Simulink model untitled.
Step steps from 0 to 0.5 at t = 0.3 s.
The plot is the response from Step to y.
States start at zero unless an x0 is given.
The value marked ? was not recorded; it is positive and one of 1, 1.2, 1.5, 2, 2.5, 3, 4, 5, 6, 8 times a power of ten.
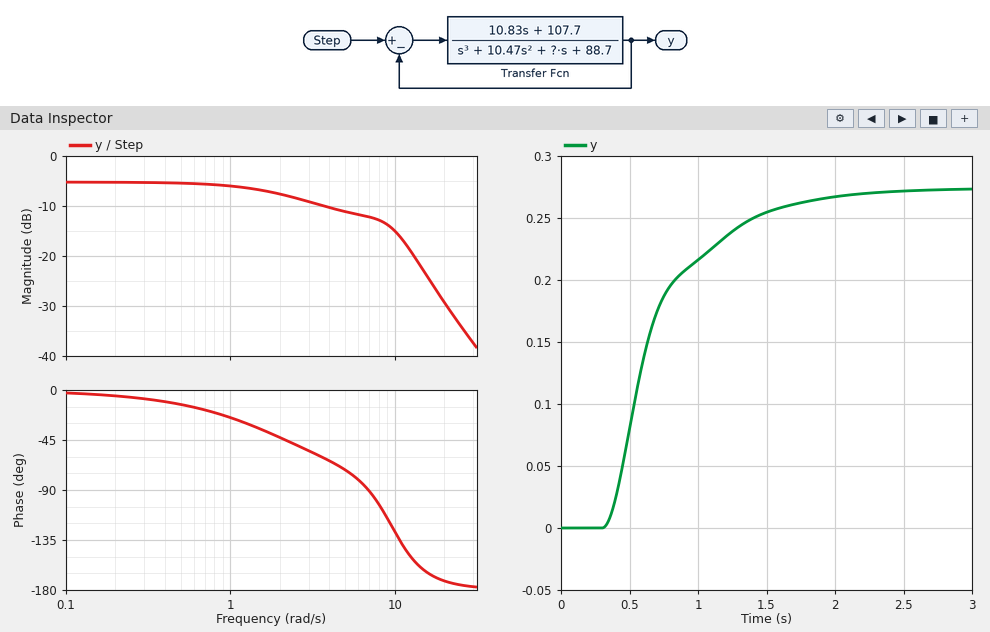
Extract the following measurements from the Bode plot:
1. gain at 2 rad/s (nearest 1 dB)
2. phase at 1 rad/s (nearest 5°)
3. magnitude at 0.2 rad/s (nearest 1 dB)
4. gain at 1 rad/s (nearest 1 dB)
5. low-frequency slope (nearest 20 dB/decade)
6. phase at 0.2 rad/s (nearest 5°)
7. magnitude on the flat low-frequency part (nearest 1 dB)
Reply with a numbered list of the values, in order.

1. -8 dB
2. -25°
3. -5 dB
4. -6 dB
5. 0 dB/decade
6. -5°
7. -5 dB
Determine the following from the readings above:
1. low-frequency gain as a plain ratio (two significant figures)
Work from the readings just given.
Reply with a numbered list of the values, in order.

1. 0.56
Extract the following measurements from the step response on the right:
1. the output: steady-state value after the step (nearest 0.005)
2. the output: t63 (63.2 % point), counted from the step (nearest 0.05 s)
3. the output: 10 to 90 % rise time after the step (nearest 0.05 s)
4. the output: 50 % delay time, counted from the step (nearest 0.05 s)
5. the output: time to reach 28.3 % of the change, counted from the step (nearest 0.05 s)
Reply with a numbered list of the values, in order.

1. 0.275
2. 0.40 s
3. 0.95 s
4. 0.30 s
5. 0.20 s
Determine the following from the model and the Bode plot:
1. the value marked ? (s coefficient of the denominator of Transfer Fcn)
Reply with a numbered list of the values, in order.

1. 100
